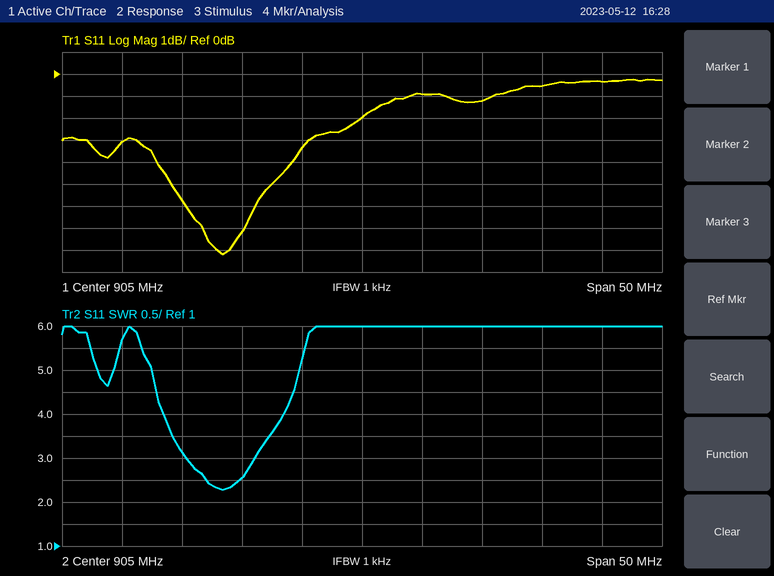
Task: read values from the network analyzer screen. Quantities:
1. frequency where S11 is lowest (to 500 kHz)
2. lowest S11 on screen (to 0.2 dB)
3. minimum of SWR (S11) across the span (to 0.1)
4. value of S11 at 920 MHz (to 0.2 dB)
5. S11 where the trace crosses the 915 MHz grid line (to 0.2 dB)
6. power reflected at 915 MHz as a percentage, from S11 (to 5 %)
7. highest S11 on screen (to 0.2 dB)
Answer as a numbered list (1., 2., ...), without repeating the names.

1. 893.5 MHz
2. -8.2 dB
3. 2.3
4. -0.6 dB
5. -1.2 dB
6. 75 %
7. -0.2 dB
